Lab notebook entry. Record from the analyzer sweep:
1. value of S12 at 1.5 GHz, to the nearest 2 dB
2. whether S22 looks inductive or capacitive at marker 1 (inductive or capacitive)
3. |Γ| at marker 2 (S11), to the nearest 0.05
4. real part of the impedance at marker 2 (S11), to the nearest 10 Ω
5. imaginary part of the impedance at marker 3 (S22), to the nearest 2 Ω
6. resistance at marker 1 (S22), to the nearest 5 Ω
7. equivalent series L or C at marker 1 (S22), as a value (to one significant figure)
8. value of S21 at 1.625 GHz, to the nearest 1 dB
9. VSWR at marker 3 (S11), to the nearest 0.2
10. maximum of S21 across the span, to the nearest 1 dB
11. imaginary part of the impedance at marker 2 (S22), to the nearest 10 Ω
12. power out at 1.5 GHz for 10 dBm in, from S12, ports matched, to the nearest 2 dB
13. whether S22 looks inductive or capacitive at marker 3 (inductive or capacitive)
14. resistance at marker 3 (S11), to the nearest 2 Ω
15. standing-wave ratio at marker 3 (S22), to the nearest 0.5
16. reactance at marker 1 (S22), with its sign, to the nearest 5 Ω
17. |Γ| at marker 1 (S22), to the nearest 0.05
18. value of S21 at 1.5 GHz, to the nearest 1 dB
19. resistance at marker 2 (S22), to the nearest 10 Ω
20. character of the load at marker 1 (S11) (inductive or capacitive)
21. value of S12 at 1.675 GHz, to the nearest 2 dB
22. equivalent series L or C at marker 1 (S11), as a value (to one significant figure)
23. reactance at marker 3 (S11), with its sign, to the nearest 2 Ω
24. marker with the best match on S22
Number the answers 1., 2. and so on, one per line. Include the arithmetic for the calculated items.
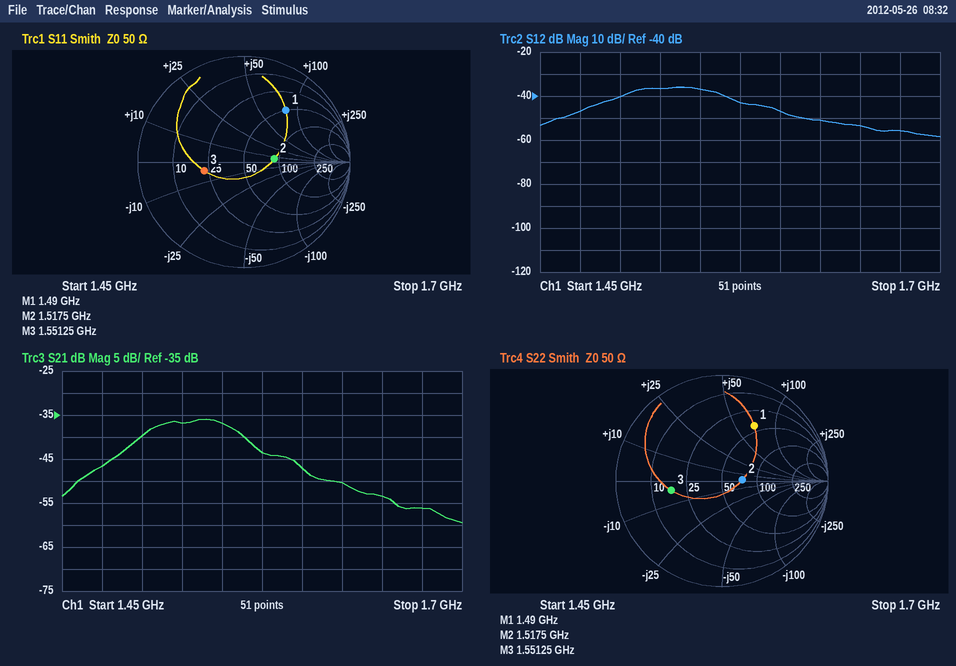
1. -40 dB
2. inductive
3. 0.30
4. 90 Ω
5. -4 Ω
6. 40 Ω
7. L = 70 Ω/(2π × 1.49 GHz) ≈ 7 nH
8. -50 dB
9. 2.2
10. -36 dB
11. 0 Ω
12. 10 dBm + (-40 dB) = -30 dBm
13. capacitive
14. 22 Ω
15. 3.0
16. +70 Ω
17. 0.60
18. -40 dB
19. 70 Ω
20. inductive
21. -56 dB
22. L = 80 Ω/(2π × 1.49 GHz) ≈ 9 nH
23. -4 Ω
24. marker 2
